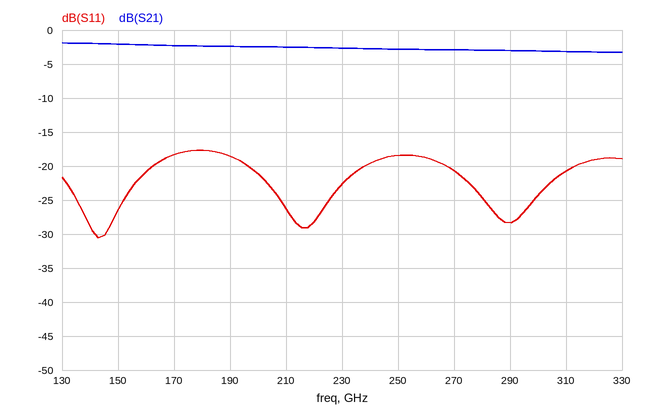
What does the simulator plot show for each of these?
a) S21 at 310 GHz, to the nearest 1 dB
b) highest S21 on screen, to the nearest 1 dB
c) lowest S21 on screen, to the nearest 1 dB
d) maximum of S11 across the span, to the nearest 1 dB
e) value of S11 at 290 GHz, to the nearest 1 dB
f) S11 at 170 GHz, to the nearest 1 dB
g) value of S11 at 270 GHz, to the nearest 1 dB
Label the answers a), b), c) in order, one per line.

a) -3 dB
b) -2 dB
c) -3 dB
d) -18 dB
e) -28 dB
f) -18 dB
g) -21 dB
